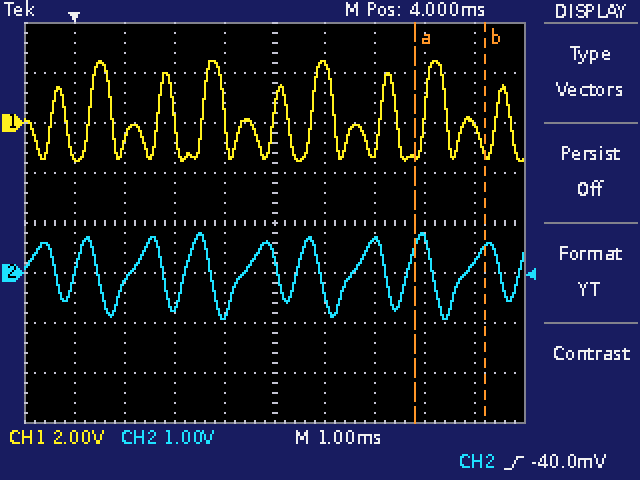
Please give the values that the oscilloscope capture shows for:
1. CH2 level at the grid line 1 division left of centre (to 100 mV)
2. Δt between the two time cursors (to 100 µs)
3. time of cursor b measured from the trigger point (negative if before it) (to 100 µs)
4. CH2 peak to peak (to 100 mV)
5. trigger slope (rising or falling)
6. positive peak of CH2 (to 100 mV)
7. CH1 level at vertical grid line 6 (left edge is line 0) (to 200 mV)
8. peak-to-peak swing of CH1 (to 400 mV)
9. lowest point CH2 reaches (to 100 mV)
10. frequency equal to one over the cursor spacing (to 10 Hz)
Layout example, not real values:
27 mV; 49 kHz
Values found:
-800 mV; 1.4 ms; +8.2 ms; 1.7 V; rising; 800 mV; 2.4 V; 4.0 V; -900 mV; 710 Hz
